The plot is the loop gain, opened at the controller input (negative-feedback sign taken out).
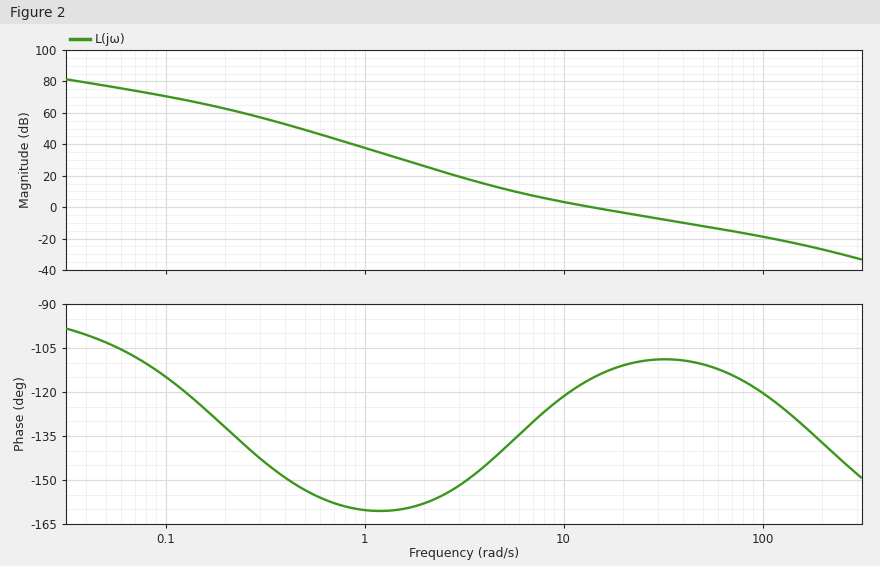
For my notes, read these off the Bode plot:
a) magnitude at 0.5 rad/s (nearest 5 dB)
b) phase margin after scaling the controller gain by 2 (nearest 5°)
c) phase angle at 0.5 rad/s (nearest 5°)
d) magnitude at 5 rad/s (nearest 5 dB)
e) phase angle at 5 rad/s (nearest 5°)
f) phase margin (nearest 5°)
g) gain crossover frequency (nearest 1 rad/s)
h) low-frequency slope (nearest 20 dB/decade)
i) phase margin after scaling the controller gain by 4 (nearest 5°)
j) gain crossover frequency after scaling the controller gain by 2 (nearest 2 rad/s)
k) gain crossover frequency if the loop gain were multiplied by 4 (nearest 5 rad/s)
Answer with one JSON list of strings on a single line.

["50 dB", "70°", "-155°", "10 dB", "-140°", "65°", "14 rad/s", "-20 dB/decade", "70°", "26 rad/s", "50 rad/s"]
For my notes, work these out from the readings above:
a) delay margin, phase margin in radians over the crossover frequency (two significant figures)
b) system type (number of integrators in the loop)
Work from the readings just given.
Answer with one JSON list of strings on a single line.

["0.081 s", "1"]
